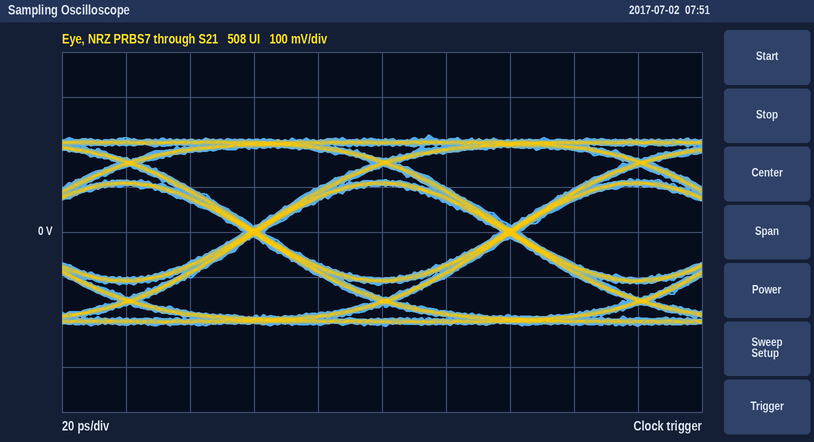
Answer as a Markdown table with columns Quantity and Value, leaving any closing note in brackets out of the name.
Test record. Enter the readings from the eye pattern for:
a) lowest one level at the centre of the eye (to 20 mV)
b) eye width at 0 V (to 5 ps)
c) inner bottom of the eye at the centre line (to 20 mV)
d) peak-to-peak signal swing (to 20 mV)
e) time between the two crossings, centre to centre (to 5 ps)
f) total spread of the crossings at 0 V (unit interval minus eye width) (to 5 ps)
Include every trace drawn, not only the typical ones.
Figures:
| Quantity | Value |
|---|---|
| lowest one level at the centre of the eye | 100 mV |
| eye width at 0 V | 75 ps |
| inner bottom of the eye at the centre line | -100 mV |
| peak-to-peak signal swing | 420 mV |
| time between the two crossings, centre to centre | 80 ps |
| total spread of the crossings at 0 V (unit interval minus eye width) | 5 ps |
